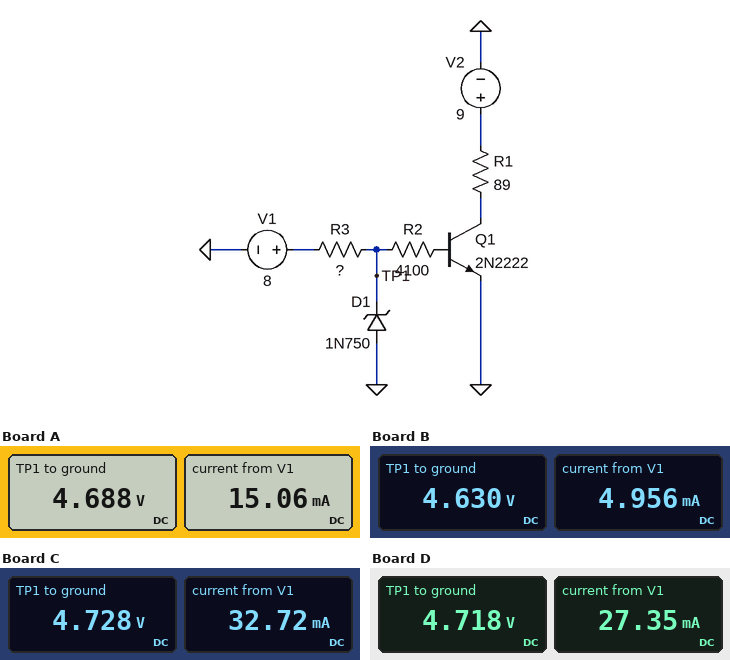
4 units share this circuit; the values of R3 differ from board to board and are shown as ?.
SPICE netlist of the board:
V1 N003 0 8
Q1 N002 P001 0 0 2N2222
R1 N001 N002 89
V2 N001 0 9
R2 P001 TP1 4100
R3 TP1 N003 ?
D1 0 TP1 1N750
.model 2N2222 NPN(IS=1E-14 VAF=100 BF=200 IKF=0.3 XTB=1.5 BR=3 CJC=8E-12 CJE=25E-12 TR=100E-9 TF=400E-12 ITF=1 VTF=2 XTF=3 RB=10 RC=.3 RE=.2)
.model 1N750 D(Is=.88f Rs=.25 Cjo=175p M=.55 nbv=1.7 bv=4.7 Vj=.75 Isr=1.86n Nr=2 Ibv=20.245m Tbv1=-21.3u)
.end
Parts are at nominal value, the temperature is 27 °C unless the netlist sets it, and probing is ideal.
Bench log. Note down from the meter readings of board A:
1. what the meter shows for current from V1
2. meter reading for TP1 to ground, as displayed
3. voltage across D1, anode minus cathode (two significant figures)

15.06 mA
4.688 V
-4.7 V
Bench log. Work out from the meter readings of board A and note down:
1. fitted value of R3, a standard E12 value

220 Ω
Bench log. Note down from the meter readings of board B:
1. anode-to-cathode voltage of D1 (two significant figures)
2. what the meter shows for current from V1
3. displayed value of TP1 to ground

-4.6 V
4.956 mA
4.630 V
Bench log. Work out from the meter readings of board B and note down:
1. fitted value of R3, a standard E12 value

680 Ω
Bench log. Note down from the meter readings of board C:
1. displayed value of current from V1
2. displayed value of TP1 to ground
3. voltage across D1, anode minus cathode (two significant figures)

32.72 mA
4.728 V
-4.7 V
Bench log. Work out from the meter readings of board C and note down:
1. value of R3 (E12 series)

100 Ω
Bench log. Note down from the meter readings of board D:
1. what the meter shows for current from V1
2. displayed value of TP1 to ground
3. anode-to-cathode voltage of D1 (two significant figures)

27.35 mA
4.718 V
-4.7 V
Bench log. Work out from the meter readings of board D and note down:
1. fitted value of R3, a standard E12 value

120 Ω
